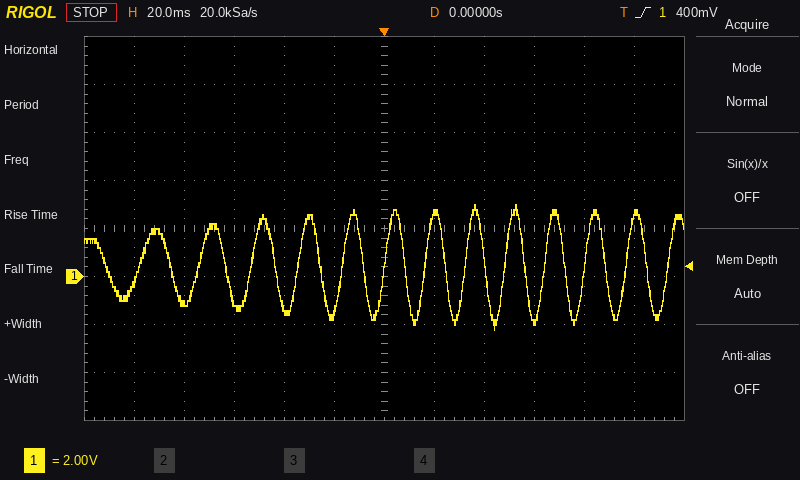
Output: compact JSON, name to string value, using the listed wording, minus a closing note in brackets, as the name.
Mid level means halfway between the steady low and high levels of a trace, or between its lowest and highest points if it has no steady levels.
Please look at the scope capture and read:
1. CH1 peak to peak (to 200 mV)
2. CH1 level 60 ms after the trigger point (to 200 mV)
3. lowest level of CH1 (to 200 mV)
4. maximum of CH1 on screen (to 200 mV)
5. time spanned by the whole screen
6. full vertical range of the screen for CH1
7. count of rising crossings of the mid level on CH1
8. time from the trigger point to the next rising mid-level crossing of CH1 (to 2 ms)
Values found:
{"CH1 peak to peak": "5.2 V", "CH1 level 60 ms after the trigger point": "-1.8 V", "lowest level of CH1": "-2.2 V", "maximum of CH1 on screen": "3.0 V", "time spanned by the whole screen": "240 ms", "full vertical range of the screen for CH1": "16 V", "count of rising crossings of the mid level on CH1": "13", "time from the trigger point to the next rising mid-level crossing of CH1": "16 ms"}
